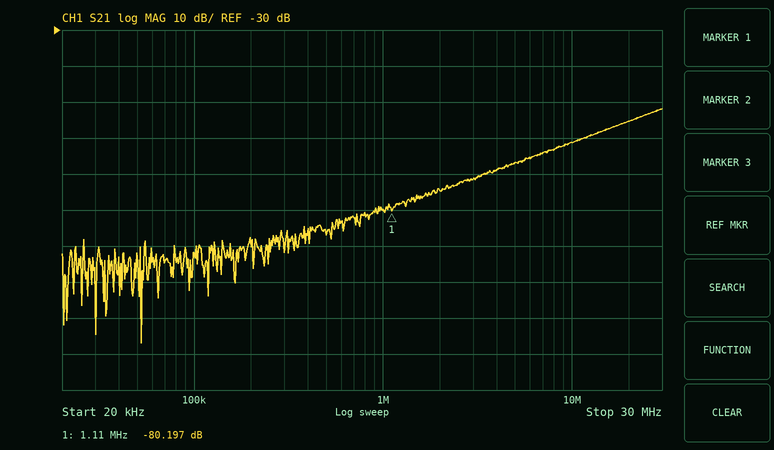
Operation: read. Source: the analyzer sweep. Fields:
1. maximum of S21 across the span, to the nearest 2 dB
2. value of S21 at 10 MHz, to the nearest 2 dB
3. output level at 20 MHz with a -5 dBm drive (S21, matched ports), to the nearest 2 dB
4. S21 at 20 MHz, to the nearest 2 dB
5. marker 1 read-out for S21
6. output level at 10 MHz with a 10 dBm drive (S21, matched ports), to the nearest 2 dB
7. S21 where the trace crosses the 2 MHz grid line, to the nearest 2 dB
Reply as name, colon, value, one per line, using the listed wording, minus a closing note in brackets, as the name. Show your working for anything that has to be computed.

maximum of S21 across the span, to the nearest 2 dB: -52 dB
value of S21 at 10 MHz, to the nearest 2 dB: -62 dB
output level at 20 MHz with a -5 dBm drive (S21, matched ports), to the nearest 2 dB: -5 dBm + (-56 dB) = -60 dBm
S21 at 20 MHz, to the nearest 2 dB: -56 dB
marker 1 read-out for S21: -80.197 dB
output level at 10 MHz with a 10 dBm drive (S21, matched ports), to the nearest 2 dB: 10 dBm + (-62 dB) = -52 dBm
S21 where the trace crosses the 2 MHz grid line, to the nearest 2 dB: -74 dB
